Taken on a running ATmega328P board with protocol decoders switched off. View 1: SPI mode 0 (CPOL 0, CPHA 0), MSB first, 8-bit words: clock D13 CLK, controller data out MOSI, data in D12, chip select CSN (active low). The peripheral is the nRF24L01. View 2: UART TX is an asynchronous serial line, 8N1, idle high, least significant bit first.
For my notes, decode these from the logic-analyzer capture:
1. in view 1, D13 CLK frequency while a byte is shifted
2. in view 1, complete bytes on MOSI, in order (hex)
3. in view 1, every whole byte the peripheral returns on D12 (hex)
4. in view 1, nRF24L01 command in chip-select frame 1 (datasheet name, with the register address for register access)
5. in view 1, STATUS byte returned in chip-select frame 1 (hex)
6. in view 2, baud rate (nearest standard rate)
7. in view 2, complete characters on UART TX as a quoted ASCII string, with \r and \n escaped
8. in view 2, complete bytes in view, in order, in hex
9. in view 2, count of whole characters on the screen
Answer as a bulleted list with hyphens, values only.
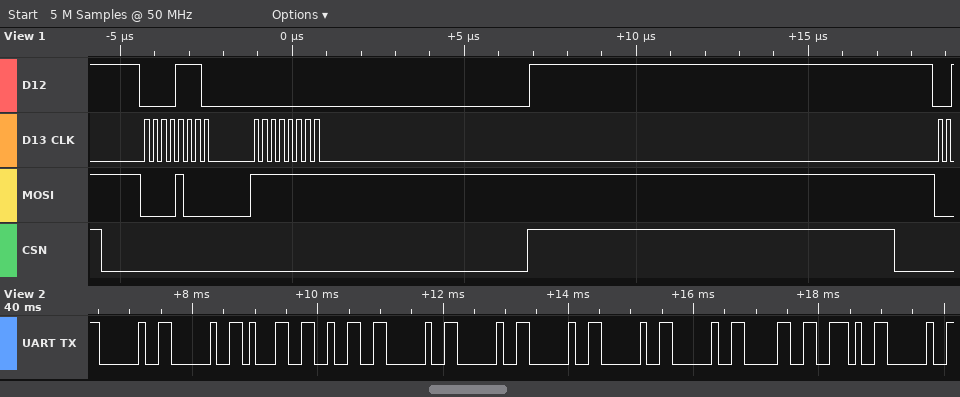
- 4 MHz
- 08 FF
- 0E 00
- R_REGISTER 0x08
- 0x0E
- 9600 baud
- "  12     0. "
- 20 20 31 32 20 20 20 20 20 30 2E 20
- 12
